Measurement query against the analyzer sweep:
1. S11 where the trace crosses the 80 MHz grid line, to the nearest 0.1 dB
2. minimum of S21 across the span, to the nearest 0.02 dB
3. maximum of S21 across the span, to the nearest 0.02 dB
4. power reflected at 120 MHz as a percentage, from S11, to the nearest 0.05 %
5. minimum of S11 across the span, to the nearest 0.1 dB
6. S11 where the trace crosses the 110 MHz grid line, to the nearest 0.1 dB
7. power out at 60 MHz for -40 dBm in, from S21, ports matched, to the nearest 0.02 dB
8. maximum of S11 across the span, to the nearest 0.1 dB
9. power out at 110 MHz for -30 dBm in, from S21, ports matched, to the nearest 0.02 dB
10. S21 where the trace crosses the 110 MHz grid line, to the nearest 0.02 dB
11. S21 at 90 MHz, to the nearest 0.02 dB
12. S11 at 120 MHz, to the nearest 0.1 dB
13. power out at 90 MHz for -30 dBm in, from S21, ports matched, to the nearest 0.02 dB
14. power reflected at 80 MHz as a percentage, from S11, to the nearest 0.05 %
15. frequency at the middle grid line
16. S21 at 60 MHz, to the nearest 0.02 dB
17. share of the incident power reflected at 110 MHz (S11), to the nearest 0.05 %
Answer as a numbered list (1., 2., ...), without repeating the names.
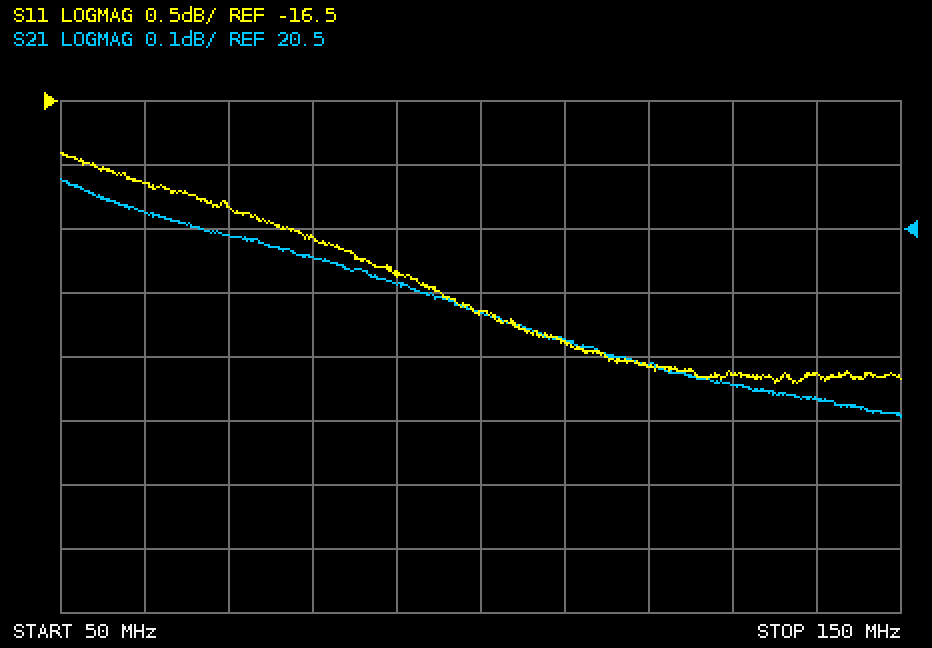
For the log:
1. -17.6 dB
2. 20.20 dB
3. 20.58 dB
4. 1.40 %
5. -18.7 dB
6. -18.4 dB
7. -19.48 dBm
8. -16.9 dB
9. -9.68 dBm
10. 20.32 dB
11. 20.42 dB
12. -18.6 dB
13. -9.58 dBm
14. 1.75 %
15. 100 MHz
16. 20.52 dB
17. 1.45 %
